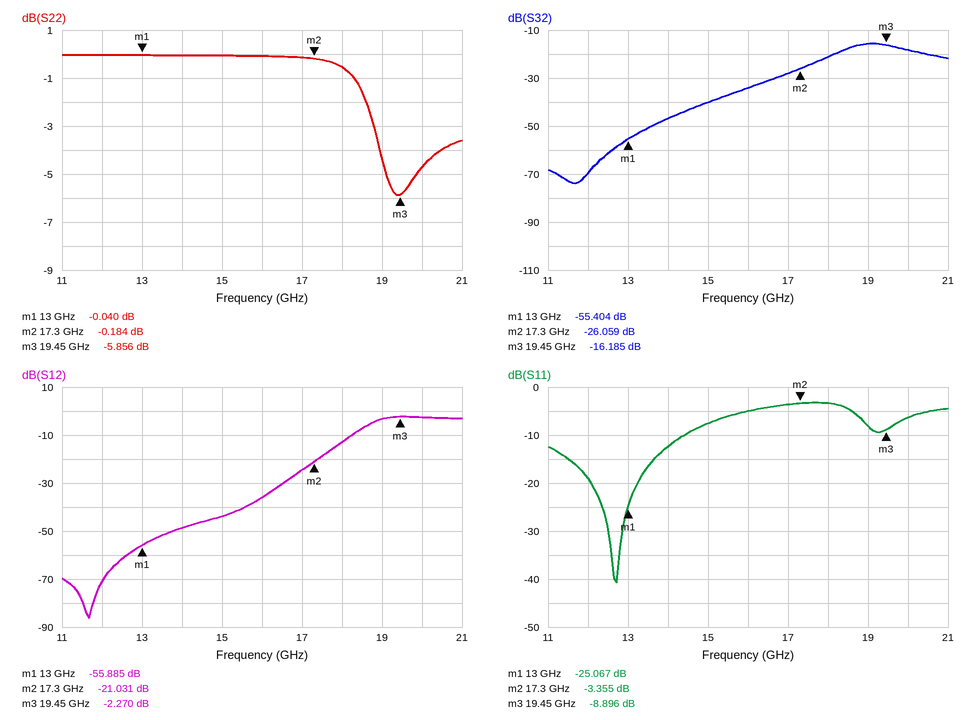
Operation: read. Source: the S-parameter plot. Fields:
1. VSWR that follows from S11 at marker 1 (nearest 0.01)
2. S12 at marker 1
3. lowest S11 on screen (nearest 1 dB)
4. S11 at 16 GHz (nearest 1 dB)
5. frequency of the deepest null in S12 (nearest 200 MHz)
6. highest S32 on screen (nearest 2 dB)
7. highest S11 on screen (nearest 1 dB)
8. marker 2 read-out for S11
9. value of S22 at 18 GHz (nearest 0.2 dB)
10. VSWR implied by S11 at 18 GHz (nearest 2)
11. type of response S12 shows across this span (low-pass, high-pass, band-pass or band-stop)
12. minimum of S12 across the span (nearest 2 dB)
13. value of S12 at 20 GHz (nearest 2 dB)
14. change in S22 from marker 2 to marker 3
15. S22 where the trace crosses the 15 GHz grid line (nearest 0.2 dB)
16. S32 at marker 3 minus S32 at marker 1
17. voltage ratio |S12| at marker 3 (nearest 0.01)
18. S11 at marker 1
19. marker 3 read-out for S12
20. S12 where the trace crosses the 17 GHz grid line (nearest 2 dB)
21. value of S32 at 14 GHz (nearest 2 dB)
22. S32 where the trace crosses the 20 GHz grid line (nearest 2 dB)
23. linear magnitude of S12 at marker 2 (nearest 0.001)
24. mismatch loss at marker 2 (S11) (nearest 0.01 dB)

1.12
-55.885 dB
-41 dB
-5 dB
11.6 GHz
-16 dB
-3 dB
-3.355 dB
-0.6 dB
6
high-pass
-86 dB
-2 dB
-5.672 dB
0.0 dB
39.219 dB
0.77
-25.067 dB
-2.270 dB
-24 dB
-46 dB
-18 dB
0.089
2.69 dB
